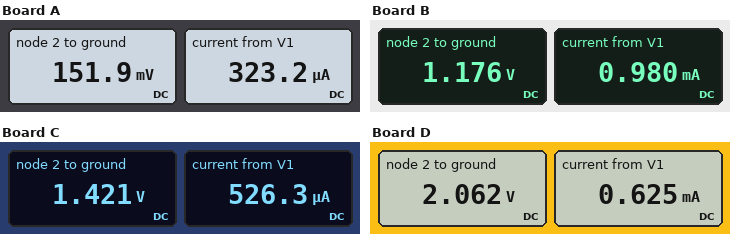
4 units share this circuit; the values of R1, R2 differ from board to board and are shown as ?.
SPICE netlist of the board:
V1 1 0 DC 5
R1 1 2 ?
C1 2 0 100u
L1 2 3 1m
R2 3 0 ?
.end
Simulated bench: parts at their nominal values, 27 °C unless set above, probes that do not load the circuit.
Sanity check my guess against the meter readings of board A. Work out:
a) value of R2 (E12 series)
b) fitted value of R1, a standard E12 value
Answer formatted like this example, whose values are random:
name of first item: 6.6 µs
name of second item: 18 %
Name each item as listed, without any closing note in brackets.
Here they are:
value of R2: 470 Ω
fitted value of R1, a standard E12 value: 15 kΩ
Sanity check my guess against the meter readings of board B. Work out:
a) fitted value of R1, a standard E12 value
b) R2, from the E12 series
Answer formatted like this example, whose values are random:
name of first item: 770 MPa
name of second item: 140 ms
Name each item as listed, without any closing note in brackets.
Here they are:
fitted value of R1, a standard E12 value: 3.9 kΩ
R2, from the E12 series: 1.2 kΩ
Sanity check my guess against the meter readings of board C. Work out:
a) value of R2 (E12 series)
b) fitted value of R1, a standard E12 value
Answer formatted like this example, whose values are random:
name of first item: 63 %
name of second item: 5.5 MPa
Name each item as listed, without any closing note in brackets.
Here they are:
value of R2: 2.7 kΩ
fitted value of R1, a standard E12 value: 6.8 kΩ
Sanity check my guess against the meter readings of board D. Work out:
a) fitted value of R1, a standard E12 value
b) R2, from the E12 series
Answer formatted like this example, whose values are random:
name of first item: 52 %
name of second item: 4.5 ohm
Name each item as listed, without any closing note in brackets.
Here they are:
fitted value of R1, a standard E12 value: 4.7 kΩ
R2, from the E12 series: 3.3 kΩ
